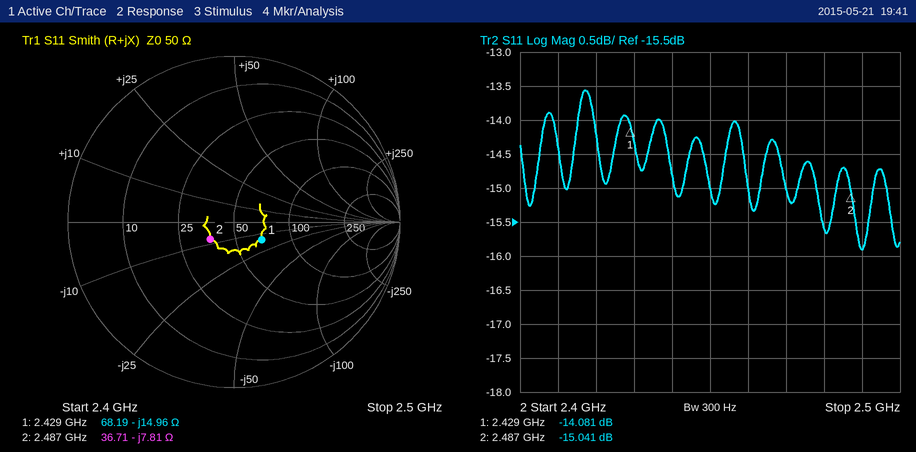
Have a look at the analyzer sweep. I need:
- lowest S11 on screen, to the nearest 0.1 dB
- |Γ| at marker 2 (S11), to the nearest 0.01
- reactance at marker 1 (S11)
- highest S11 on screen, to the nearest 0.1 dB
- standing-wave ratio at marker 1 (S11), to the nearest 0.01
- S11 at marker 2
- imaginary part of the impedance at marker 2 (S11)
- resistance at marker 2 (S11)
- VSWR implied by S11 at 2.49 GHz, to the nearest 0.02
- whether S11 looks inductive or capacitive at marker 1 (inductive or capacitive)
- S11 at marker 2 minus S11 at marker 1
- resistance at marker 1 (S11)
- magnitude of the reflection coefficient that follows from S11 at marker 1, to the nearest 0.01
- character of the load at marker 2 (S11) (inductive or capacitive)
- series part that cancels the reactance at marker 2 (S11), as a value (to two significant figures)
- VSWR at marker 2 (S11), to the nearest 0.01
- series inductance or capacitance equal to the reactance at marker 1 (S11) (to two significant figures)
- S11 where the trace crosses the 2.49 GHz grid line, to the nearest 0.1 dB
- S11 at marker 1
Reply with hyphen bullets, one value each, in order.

- -15.9 dB
- 0.18
- -14.96 Ω
- -13.6 dB
- 1.49
- -15.041 dB
- -7.81 Ω
- 36.71 Ω
- 1.38
- capacitive
- -0.960 dB
- 68.19 Ω
- 0.20
- capacitive
- 500 pH
- 1.43
- 4.4 pF
- -15.9 dB
- -14.081 dB
